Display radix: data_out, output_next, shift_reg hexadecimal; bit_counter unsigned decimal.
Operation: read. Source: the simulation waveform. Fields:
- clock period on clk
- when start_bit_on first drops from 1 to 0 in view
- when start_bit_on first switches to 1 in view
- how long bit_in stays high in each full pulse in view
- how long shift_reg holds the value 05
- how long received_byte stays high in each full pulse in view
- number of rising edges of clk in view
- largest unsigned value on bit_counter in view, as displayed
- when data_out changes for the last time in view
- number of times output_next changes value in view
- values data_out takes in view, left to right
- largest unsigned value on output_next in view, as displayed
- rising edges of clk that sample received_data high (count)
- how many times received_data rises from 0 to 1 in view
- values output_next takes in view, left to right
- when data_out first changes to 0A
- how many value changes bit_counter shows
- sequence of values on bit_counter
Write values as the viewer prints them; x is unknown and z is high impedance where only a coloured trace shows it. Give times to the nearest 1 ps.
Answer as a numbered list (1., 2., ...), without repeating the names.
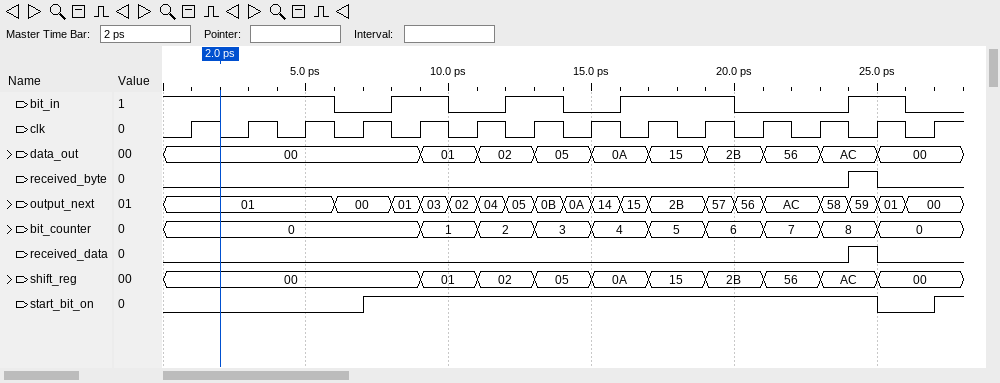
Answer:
1. 2 ps
2. 25 ps
3. 7 ps
4. 2 ps, 2 ps, 4 ps, 2 ps
5. 2 ps
6. 1 ps
7. 14
8. 8
9. 25 ps
10. 18
11. 00, 01, 02, 05, 0A, 15, 2B, 56, AC, 00
12. AC
13. 1
14. 1
15. 01, 00, 01, 03, 02, 04, 05, 0B, 0A, 14, 15, 2B, 57, 56, AC, 58, 59, 01, 00
16. 15 ps
17. 9
18. 0, 1, 2, 3, 4, 5, 6, 7, 8, 0
